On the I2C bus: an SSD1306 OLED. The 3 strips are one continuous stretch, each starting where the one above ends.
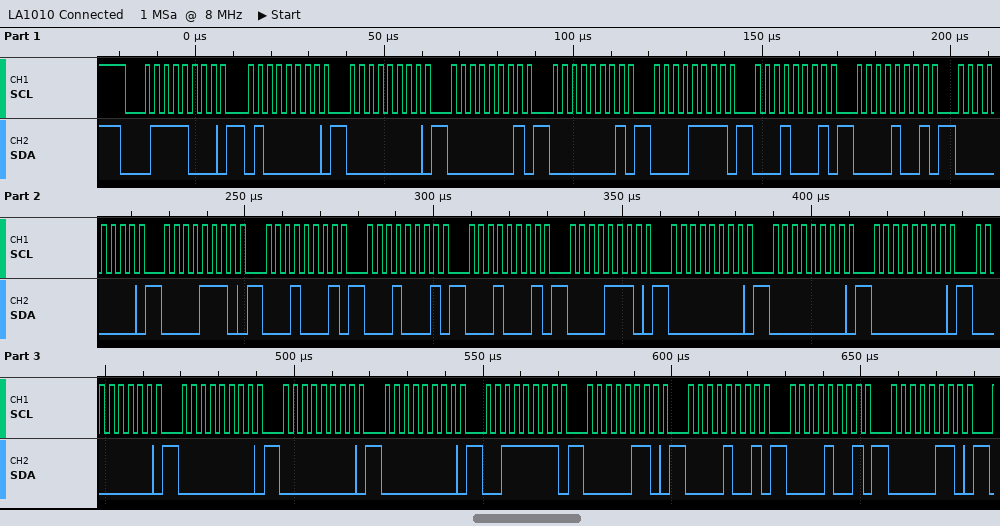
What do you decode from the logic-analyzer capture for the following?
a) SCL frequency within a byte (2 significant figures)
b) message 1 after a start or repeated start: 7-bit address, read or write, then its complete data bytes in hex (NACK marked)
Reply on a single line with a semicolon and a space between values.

400 kHz; 0x3C write: 40 00 01 01 0F 11 09 00 0E 11 11 11 0E 00 00 00 00 00 00 00 3F 06 09 09 06
